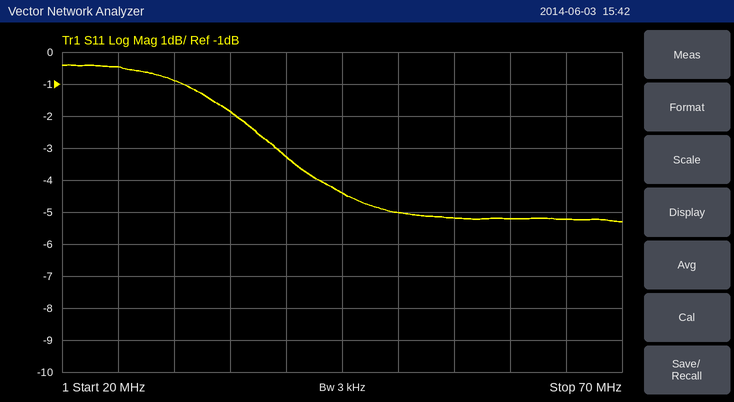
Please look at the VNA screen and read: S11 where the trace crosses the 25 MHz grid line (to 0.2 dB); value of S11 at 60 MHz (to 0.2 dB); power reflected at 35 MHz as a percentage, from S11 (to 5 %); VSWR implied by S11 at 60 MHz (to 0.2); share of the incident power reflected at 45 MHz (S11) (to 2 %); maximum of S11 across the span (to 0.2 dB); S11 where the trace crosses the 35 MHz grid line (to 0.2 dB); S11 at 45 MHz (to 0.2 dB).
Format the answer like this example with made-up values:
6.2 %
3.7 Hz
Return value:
-0.4 dB
-5.2 dB
65 %
3.4
36 %
-0.4 dB
-1.8 dB
-4.4 dB
